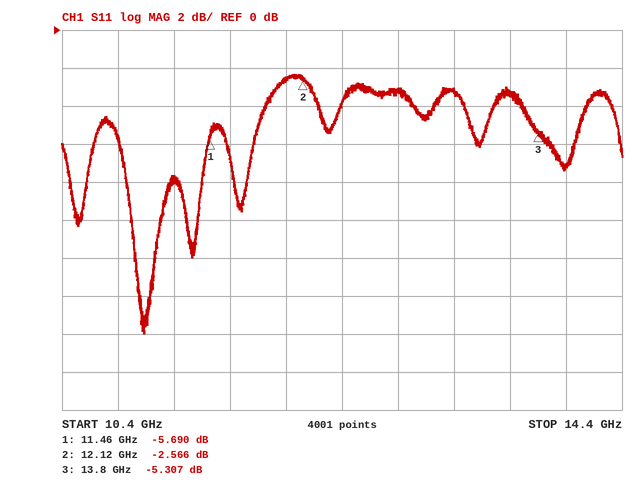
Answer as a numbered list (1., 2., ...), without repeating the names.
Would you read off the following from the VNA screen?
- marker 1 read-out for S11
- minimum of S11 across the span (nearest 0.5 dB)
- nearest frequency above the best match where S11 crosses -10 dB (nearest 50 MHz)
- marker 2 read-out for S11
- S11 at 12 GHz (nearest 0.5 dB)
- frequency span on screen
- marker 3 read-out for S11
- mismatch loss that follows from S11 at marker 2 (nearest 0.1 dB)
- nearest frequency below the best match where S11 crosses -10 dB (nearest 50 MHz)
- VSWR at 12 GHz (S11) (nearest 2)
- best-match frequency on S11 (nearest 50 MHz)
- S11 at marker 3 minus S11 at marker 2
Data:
1. -5.690 dB
2. -16.0 dB
3. 11.10 GHz
4. -2.566 dB
5. -2.5 dB
6. 4 GHz
7. -5.307 dB
8. 3.5 dB
9. 10.90 GHz
10. 6
11. 11.00 GHz
12. -2.741 dB
